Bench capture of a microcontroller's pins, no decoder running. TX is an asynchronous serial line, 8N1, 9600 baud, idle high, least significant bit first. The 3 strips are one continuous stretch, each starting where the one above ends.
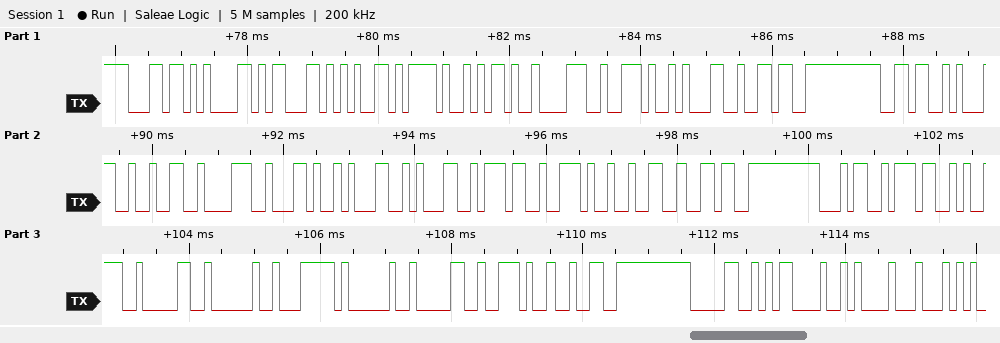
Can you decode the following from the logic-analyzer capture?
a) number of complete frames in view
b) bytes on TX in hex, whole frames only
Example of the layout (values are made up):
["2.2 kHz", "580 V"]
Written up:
["35", "6C 61 63 65 2F 2D 38 2E 31 36 36 31 32 38 2C 31 31 37 2E 32 36 34 37 39 30 20 7C 20 30 2E 32 30 0D 0A 44"]
